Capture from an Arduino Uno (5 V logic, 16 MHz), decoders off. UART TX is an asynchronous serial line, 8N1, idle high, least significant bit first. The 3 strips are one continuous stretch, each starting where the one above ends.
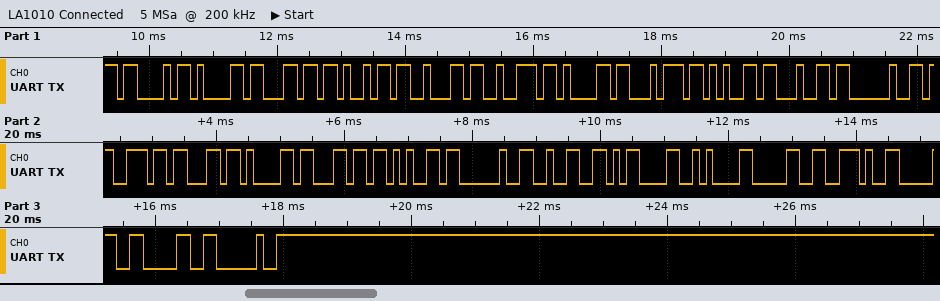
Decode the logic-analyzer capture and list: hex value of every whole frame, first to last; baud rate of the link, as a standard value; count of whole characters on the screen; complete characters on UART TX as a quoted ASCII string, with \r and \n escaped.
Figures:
43 61 6C 69 62 72 61 74 65 64 20 73 63 61 6C 65 20 32 0D 0A 30 2E 30 30 20
9600 baud
25
"Calibrated scale 2\r\n0.00 "
